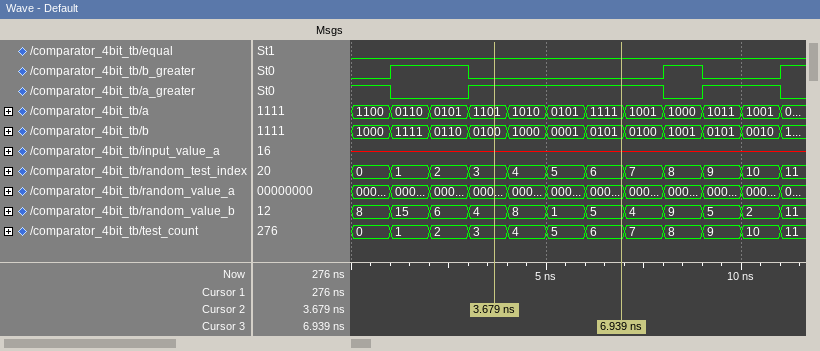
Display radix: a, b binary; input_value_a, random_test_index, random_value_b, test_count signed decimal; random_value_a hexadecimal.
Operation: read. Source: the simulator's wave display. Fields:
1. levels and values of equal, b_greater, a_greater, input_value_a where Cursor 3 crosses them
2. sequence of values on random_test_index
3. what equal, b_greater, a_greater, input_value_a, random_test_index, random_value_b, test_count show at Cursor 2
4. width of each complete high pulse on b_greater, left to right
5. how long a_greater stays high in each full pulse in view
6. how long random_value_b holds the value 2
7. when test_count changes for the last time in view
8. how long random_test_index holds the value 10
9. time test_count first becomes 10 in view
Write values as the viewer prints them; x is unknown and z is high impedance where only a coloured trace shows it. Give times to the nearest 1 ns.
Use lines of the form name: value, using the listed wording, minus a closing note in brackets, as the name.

levels and values of equal, b_greater, a_greater, input_value_a where Cursor 3 crosses them: equal=0, b_greater=0, a_greater=1, input_value_a=x
sequence of values on random_test_index: 0, 1, 2, 3, 4, 5, 6, 7, 8, 9, 10, 11
what equal, b_greater, a_greater, input_value_a, random_test_index, random_value_b, test_count show at Cursor 2: equal=0, b_greater=0, a_greater=1, input_value_a=x, random_test_index=3, random_value_b=4, test_count=3
width of each complete high pulse on b_greater, left to right: 2 ns, 1 ns
how long a_greater stays high in each full pulse in view: 5 ns, 2 ns
how long random_value_b holds the value 2: 1 ns
when test_count changes for the last time in view: 11 ns
how long random_test_index holds the value 10: 1 ns
time test_count first becomes 10 in view: 10 ns
